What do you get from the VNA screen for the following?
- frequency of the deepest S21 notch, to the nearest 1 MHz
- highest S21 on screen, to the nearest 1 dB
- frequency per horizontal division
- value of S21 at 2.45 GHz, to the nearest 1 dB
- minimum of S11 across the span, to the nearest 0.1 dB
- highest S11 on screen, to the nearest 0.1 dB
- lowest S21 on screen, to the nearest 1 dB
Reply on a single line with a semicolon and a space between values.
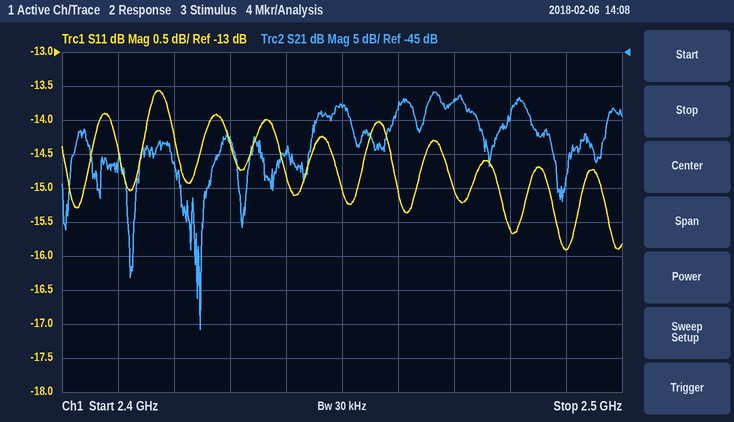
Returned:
2.425 GHz; -51 dB; 10 MHz; -53 dB; -15.9 dB; -13.6 dB; -86 dB
